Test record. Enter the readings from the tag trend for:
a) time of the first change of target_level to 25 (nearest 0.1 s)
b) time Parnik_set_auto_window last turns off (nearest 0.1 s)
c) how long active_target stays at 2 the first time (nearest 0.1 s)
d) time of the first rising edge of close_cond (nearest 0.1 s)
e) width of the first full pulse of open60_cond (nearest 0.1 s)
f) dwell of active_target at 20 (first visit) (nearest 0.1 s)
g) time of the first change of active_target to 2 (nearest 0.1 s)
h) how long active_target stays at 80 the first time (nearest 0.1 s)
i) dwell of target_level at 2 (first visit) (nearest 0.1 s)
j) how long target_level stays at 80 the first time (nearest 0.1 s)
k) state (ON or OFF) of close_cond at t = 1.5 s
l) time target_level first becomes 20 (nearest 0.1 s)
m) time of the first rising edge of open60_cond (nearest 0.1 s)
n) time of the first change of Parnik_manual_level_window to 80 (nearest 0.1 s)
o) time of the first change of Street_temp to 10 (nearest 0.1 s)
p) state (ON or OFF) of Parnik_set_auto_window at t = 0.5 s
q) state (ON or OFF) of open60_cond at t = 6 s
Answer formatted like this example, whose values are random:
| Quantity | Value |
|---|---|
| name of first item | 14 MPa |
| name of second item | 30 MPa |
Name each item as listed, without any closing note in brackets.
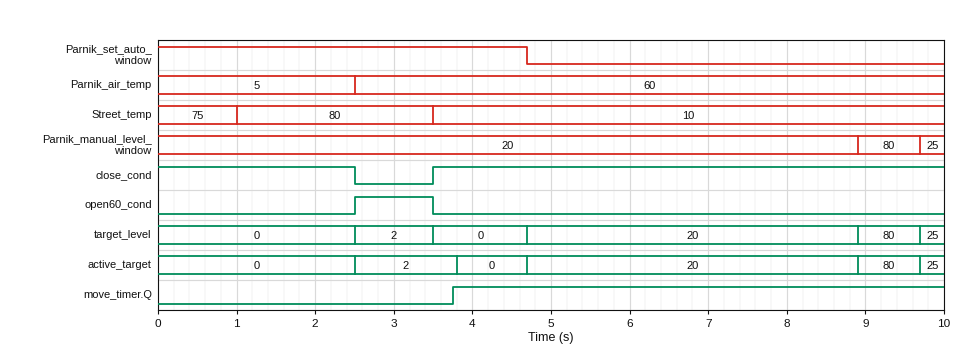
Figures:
| Quantity | Value |
|---|---|
| time of the first change of target_level to 25 | 9.7 s |
| time Parnik_set_auto_window last turns off | 4.7 s |
| how long active_target stays at 2 the first time | 1.3 s |
| time of the first rising edge of close_cond | 3.5 s |
| width of the first full pulse of open60_cond | 1.0 s |
| dwell of active_target at 20 (first visit) | 4.2 s |
| time of the first change of active_target to 2 | 2.5 s |
| how long active_target stays at 80 the first time | 0.8 s |
| dwell of target_level at 2 (first visit) | 1.0 s |
| how long target_level stays at 80 the first time | 0.8 s |
| state (ON or OFF) of close_cond at t = 1.5 s | ON |
| time target_level first becomes 20 | 4.7 s |
| time of the first rising edge of open60_cond | 2.5 s |
| time of the first change of Parnik_manual_level_window to 80 | 8.9 s |
| time of the first change of Street_temp to 10 | 3.5 s |
| state (ON or OFF) of Parnik_set_auto_window at t = 0.5 s | ON |
| state (ON or OFF) of open60_cond at t = 6 s | OFF |
